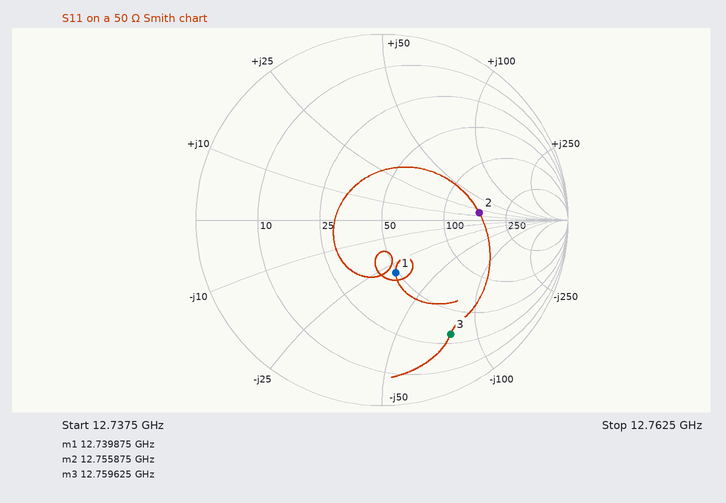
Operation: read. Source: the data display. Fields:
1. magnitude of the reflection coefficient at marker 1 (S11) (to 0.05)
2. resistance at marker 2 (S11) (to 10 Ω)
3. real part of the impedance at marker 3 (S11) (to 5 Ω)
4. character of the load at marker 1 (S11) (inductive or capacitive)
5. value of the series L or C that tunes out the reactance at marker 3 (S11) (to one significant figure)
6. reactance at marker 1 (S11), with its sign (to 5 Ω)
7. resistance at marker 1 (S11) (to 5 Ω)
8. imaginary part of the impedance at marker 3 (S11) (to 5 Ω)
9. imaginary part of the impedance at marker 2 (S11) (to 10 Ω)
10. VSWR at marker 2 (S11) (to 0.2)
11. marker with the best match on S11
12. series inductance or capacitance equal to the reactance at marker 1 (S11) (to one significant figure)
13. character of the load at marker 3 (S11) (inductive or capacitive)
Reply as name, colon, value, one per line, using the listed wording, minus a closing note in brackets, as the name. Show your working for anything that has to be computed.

magnitude of the reflection coefficient at marker 1 (S11): 0.30
resistance at marker 2 (S11): 160 Ω
real part of the impedance at marker 3 (S11): 30 Ω
character of the load at marker 1 (S11): capacitive
value of the series L or C that tunes out the reactance at marker 3 (S11): L = 80 Ω/(2π × 12.759625 GHz) ≈ 1.0 nH
reactance at marker 1 (S11), with its sign: -30 Ω
resistance at marker 1 (S11): 50 Ω
imaginary part of the impedance at marker 3 (S11): -80 Ω
imaginary part of the impedance at marker 2 (S11): +20 Ω
VSWR at marker 2 (S11): 3.2
marker with the best match on S11: marker 1
series inductance or capacitance equal to the reactance at marker 1 (S11): C = 1/(2π × 12.739875 GHz × 30 Ω) ≈ 416 fF, so 400 fF to one significant figure
character of the load at marker 3 (S11): capacitive
